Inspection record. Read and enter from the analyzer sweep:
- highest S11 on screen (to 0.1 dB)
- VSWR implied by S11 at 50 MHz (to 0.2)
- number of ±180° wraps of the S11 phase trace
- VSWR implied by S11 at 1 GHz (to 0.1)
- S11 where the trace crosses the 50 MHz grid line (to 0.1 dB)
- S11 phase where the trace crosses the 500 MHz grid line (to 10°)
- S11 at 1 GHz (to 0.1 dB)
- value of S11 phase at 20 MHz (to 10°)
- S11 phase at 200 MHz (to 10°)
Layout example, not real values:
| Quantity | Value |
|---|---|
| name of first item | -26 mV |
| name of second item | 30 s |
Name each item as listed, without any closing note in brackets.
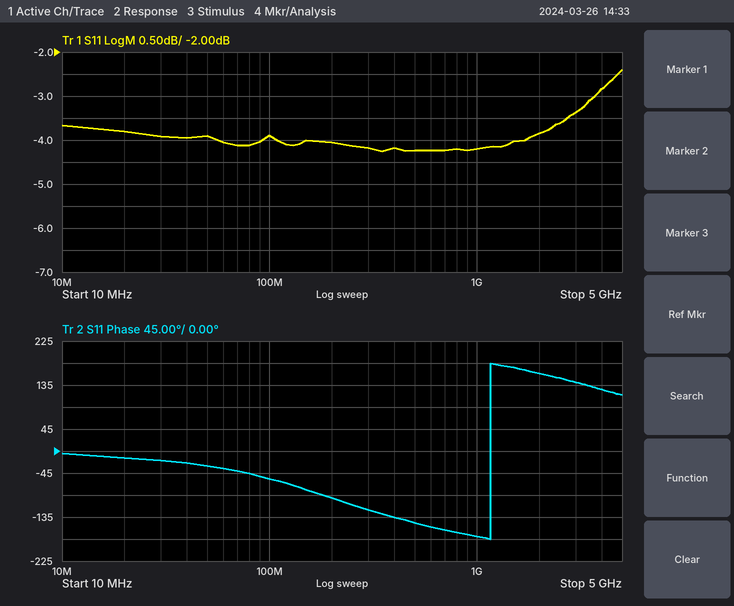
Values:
| Quantity | Value |
|---|---|
| highest S11 on screen | -2.4 dB |
| VSWR implied by S11 at 50 MHz | 4.6 |
| number of ±180° wraps of the S11 phase trace | 1 |
| VSWR implied by S11 at 1 GHz | 4.2 |
| S11 where the trace crosses the 50 MHz grid line | -3.9 dB |
| S11 phase where the trace crosses the 500 MHz grid line | -150° |
| S11 at 1 GHz | -4.2 dB |
| value of S11 phase at 20 MHz | -10° |
| S11 phase at 200 MHz | -100° |
